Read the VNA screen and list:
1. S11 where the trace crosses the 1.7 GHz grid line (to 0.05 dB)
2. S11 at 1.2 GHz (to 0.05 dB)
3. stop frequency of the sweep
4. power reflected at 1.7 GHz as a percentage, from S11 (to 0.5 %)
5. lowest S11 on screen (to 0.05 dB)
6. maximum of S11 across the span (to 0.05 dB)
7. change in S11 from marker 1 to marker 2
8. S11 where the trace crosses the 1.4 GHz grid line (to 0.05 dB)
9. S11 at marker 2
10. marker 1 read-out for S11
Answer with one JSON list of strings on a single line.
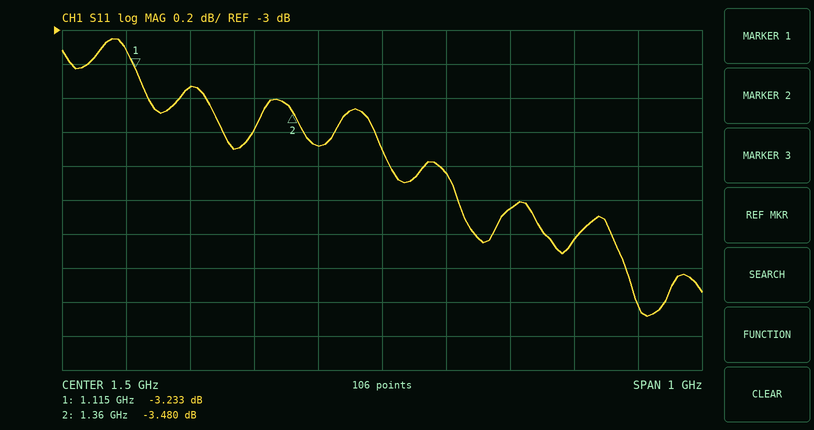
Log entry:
["-4.05 dB", "-3.35 dB", "2 GHz", "39.5 %", "-4.70 dB", "-3.05 dB", "-0.247 dB", "-3.70 dB", "-3.480 dB", "-3.233 dB"]
